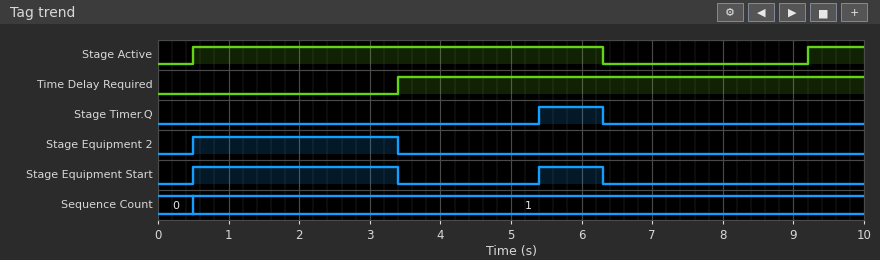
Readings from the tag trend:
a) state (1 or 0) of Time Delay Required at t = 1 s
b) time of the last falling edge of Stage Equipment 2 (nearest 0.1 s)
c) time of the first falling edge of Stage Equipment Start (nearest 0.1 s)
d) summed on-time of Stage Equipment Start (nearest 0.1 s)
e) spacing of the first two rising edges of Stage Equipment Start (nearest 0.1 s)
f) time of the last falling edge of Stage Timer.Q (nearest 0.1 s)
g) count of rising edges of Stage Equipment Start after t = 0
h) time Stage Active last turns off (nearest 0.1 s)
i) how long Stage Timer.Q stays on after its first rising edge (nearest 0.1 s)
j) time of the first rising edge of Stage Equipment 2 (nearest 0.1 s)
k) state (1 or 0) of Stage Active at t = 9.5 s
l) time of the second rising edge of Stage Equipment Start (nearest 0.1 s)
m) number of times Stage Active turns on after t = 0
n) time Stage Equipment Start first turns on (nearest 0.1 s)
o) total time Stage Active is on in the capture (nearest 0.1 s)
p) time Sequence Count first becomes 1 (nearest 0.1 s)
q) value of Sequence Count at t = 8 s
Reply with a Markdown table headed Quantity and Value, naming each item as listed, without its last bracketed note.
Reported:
| Quantity | Value |
|---|---|
| state (1 or 0) of Time Delay Required at t = 1 s | 0 |
| time of the last falling edge of Stage Equipment 2 | 3.4 s |
| time of the first falling edge of Stage Equipment Start | 3.4 s |
| summed on-time of Stage Equipment Start | 3.8 s |
| spacing of the first two rising edges of Stage Equipment Start | 4.9 s |
| time of the last falling edge of Stage Timer.Q | 6.3 s |
| count of rising edges of Stage Equipment Start after t = 0 | 2 |
| time Stage Active last turns off | 6.3 s |
| how long Stage Timer.Q stays on after its first rising edge | 0.9 s |
| time of the first rising edge of Stage Equipment 2 | 0.5 s |
| state (1 or 0) of Stage Active at t = 9.5 s | 1 |
| time of the second rising edge of Stage Equipment Start | 5.4 s |
| number of times Stage Active turns on after t = 0 | 2 |
| time Stage Equipment Start first turns on | 0.5 s |
| total time Stage Active is on in the capture | 6.6 s |
| time Sequence Count first becomes 1 | 0.5 s |
| value of Sequence Count at t = 8 s | 1 |
